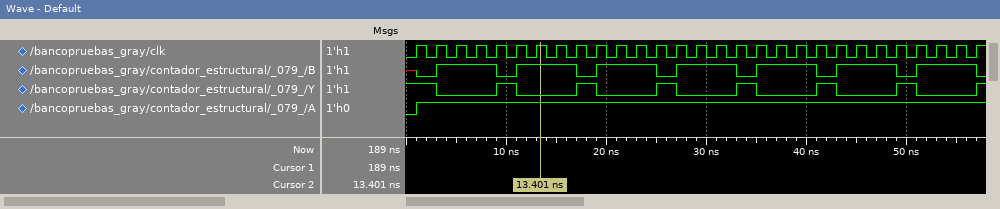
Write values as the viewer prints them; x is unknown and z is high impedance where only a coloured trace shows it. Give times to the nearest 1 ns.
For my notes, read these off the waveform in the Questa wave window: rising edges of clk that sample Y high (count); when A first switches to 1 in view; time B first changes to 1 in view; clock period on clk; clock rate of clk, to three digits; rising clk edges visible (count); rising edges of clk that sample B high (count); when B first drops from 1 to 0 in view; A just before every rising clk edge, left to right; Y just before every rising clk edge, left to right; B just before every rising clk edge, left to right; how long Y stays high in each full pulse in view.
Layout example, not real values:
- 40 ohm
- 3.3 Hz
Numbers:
- 8
- 1 ns
- 3 ns
- 2 ns
- 500 MHz
- 29
- 21
- 9 ns
- 0 1 1 1 1 1 1 1 1 1 1 1 1 1 1 1 1 1 1 1 1 1 1 1 1 1 1 1 1
- 1 1 0 0 0 1 0 0 0 1 0 0 0 1 0 0 0 1 0 0 0 1 0 0 0 1 0 0 0
- x 0 1 1 1 0 1 1 1 0 1 1 1 0 1 1 1 0 1 1 1 0 1 1 1 0 1 1 1
- 2 ns, 2 ns, 2 ns, 2 ns, 2 ns, 2 ns
